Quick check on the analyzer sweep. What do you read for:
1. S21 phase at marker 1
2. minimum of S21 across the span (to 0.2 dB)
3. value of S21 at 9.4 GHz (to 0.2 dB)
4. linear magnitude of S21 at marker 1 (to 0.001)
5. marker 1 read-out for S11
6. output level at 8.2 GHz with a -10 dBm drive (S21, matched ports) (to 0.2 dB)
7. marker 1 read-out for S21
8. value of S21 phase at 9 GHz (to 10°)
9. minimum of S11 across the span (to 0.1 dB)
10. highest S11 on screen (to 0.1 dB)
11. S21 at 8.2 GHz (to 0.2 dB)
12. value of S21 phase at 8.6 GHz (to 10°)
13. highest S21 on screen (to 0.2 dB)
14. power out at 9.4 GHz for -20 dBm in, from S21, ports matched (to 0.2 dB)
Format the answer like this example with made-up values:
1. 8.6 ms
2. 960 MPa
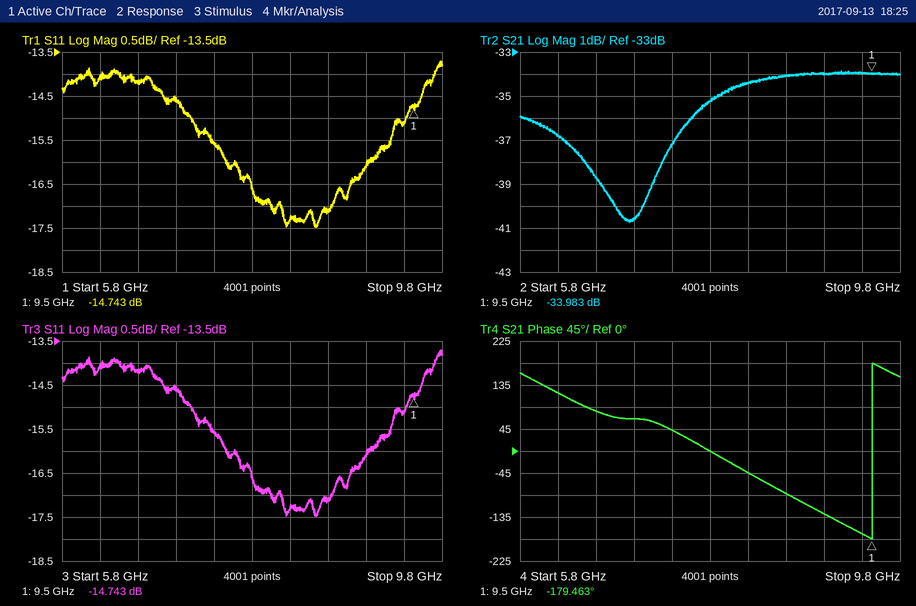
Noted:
1. -179.463°
2. -40.8 dB
3. -34.0 dB
4. 0.020
5. -14.743 dB
6. -44.4 dBm
7. -33.983 dB
8. -130°
9. -17.5 dB
10. -13.7 dB
11. -34.4 dB
12. -90°
13. -33.8 dB
14. -54.0 dBm
